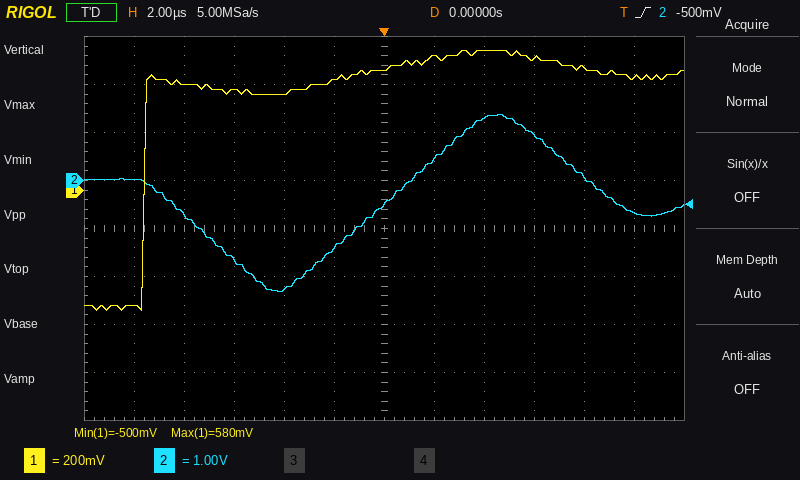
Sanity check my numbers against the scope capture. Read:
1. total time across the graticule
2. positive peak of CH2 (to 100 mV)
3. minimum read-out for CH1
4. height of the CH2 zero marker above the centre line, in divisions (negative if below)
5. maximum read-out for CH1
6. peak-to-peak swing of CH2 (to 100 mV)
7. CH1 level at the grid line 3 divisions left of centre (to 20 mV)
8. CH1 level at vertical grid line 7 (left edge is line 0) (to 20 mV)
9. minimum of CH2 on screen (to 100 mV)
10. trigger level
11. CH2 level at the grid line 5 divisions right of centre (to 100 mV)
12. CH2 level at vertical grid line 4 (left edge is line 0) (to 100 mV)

24 µs
1.4 V
-500 mV
+1.0 div
580 mV
3.7 V
420 mV
560 mV
-2.3 V
-500 mV
-700 mV
-2.3 V
